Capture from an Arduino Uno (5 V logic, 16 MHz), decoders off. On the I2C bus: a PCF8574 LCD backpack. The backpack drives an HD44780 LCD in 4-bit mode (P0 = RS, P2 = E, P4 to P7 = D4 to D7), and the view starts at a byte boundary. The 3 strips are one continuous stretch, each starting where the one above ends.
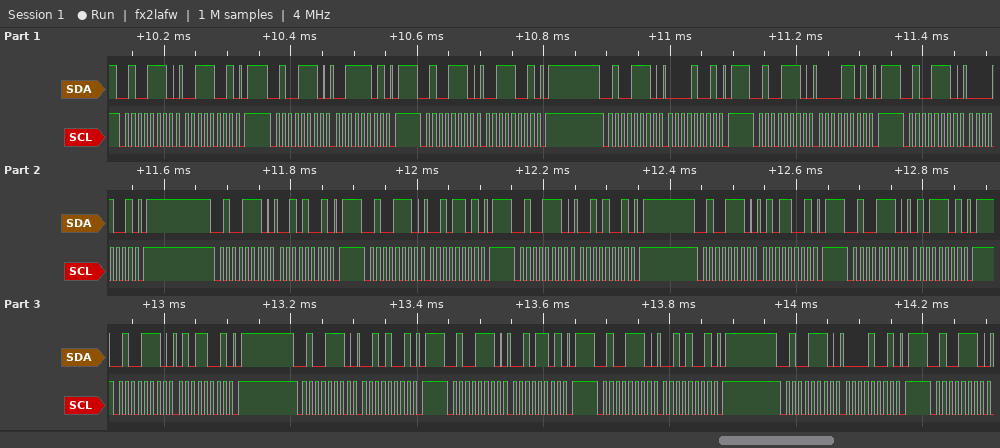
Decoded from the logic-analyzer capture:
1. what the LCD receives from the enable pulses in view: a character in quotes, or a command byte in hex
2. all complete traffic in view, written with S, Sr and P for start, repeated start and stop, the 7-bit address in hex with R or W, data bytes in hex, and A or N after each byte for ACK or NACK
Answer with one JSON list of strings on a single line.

["'0' '%'", "S 27W A 39 A P S 27W A 3D A P S 27W A 39 A P S 27W A 09 A P S 27W A 0D A P S 27W A 09 A P S 27W A 29 A P S 27W A 2D A P S 27W A 29 A P S 27W A 59 A P S 27W A 5D A P S 27W A 59 A P S 27W A 29 A P S 27W A 2D A P S 27W A 29 A P S 27W A 09 A P S 27W A"]
